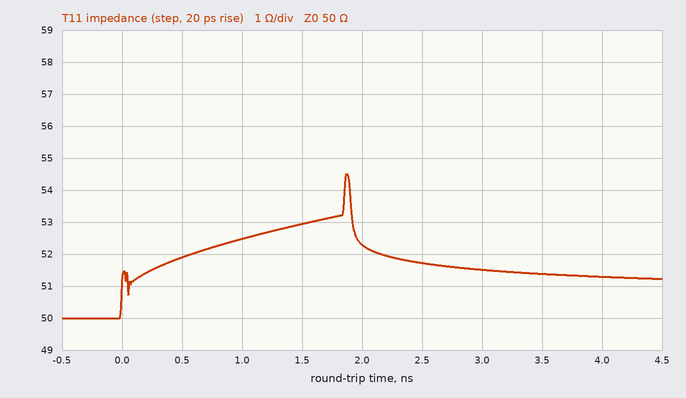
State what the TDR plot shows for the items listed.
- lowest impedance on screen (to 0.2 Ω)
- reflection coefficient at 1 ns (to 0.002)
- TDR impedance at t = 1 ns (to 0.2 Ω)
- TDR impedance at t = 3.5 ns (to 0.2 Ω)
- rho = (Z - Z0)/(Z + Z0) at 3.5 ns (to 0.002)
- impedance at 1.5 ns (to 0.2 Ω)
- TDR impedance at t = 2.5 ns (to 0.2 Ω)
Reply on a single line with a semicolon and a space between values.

50.0 Ω; +0.024; 52.4 Ω; 51.4 Ω; +0.014; 53.0 Ω; 51.8 Ω
